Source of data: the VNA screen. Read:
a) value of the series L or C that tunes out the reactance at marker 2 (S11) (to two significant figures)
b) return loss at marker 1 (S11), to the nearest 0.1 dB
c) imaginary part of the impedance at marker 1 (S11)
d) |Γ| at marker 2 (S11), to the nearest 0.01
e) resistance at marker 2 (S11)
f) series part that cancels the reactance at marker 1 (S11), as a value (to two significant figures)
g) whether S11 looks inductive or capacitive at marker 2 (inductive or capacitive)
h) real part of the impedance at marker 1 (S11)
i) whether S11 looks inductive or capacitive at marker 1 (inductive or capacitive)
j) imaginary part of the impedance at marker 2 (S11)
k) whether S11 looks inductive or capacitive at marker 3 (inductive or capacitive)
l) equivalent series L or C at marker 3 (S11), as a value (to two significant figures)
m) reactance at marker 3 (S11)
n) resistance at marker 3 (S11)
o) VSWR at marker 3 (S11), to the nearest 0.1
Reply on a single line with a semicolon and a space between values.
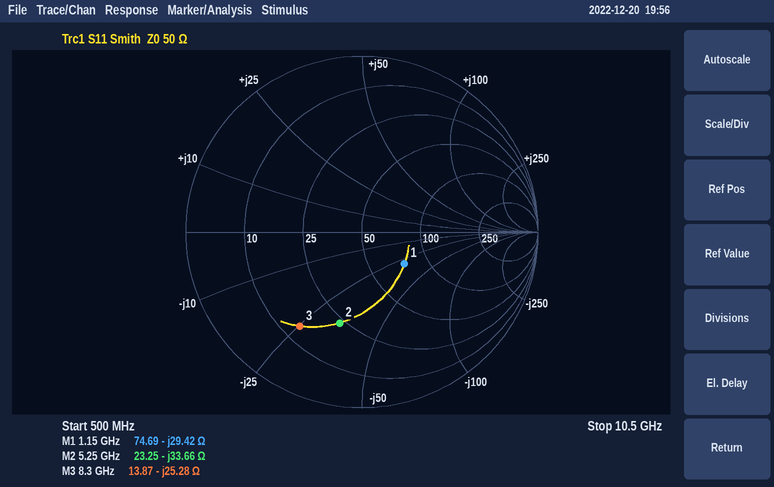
1.0 nH; 10.5 dB; -29.42 Ω; 0.53; 23.25 Ω; 4.1 nH; capacitive; 74.69 Ω; capacitive; -33.66 Ω; capacitive; 760 fF; -25.28 Ω; 13.87 Ω; 4.6
